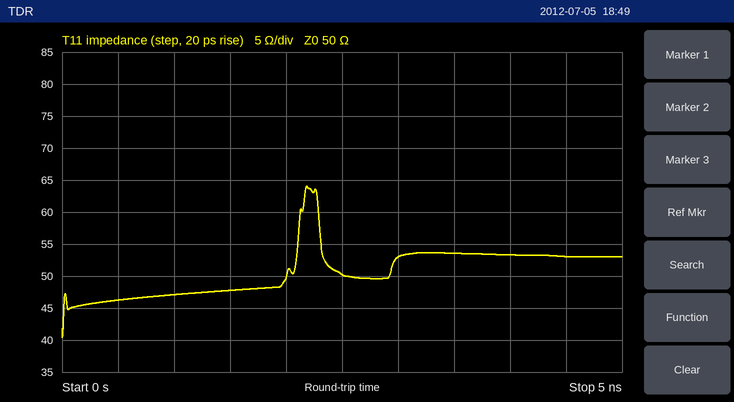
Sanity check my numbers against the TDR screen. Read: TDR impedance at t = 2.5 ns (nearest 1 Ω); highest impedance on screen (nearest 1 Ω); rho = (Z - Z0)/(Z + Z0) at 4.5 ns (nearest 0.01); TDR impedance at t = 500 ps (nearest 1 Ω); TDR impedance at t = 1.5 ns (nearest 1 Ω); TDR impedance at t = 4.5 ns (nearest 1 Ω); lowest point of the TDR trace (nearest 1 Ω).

50 Ω
64 Ω
+0.03
46 Ω
48 Ω
53 Ω
40 Ω
